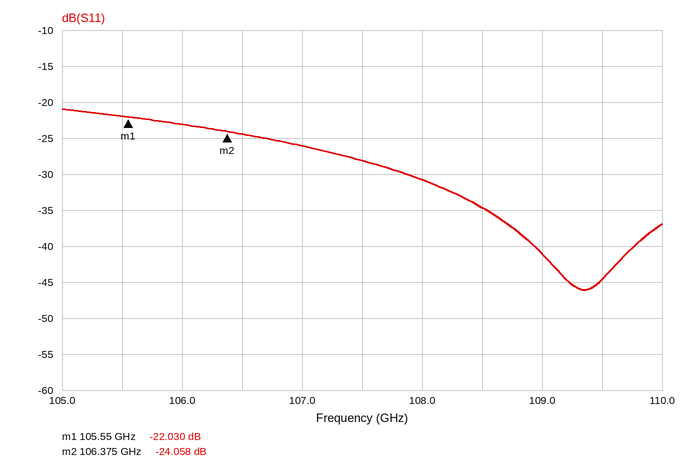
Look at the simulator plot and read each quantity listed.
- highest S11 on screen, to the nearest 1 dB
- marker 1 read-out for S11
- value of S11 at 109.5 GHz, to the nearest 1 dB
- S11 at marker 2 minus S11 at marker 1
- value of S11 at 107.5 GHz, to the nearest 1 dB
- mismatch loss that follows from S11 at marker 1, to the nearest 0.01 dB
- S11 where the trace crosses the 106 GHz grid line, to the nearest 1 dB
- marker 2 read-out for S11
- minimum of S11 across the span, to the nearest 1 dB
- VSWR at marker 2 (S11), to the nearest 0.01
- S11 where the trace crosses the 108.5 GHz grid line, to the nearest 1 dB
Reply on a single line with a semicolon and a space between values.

-21 dB; -22.030 dB; -45 dB; -2.028 dB; -28 dB; 0.03 dB; -23 dB; -24.058 dB; -46 dB; 1.13; -35 dB
